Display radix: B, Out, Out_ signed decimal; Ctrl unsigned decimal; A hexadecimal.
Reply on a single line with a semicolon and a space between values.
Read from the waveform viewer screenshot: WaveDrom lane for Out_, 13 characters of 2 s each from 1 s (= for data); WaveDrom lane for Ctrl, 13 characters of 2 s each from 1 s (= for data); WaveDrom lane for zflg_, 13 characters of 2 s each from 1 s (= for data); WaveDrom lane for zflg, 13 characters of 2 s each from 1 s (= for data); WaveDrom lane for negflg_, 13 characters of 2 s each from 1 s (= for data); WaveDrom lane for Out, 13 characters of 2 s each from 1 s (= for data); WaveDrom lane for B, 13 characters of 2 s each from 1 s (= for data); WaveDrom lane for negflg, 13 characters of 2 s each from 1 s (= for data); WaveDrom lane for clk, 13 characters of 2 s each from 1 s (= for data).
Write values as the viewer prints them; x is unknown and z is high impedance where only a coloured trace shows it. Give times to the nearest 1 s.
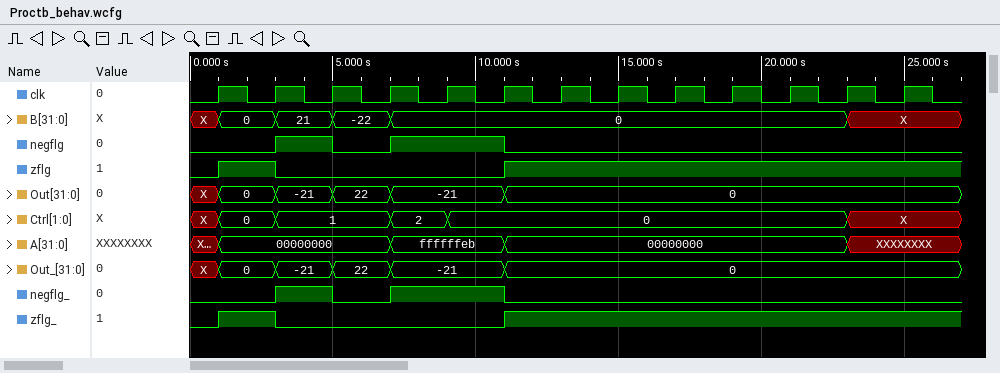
{name: 'Out_', wave: '====.=.......', data: '0 -21 22 -21 0'}; {name: 'Ctrl', wave: '==.==......x.', data: '0 1 2 0'}; {name: 'zflg_', wave: '10...1.......'}; {name: 'zflg', wave: '10...1.......'}; {name: 'negflg_', wave: '0101.0.......'}; {name: 'Out', wave: '====.=.......', data: '0 -21 22 -21 0'}; {name: 'B', wave: '====.......x.', data: '0 21 -22 0'}; {name: 'negflg', wave: '0101.0.......'}; {name: 'clk', wave: 'p............'}
